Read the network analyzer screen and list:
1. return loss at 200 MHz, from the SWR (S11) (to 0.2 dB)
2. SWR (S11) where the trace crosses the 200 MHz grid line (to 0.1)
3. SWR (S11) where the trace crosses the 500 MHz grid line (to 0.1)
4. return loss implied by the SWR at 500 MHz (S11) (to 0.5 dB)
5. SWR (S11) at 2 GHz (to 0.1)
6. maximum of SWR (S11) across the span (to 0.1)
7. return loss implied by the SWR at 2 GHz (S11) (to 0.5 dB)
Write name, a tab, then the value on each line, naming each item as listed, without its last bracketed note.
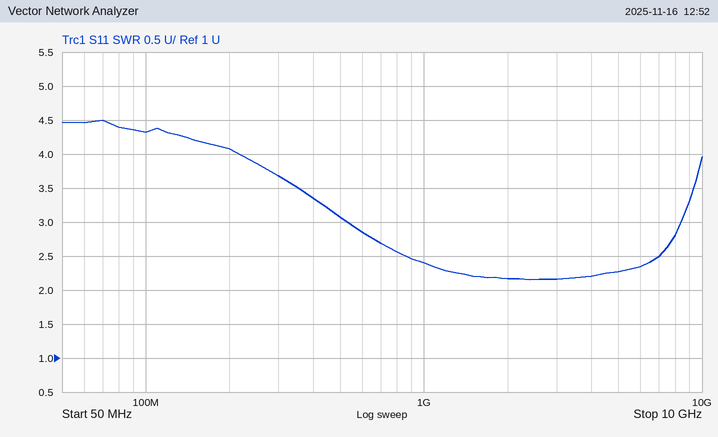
return loss at 200 MHz, from the SWR (S11)	4.4 dB
SWR (S11) where the trace crosses the 200 MHz grid line	4.1
SWR (S11) where the trace crosses the 500 MHz grid line	3.1
return loss implied by the SWR at 500 MHz (S11)	6.0 dB
SWR (S11) at 2 GHz	2.2
maximum of SWR (S11) across the span	4.5
return loss implied by the SWR at 2 GHz (S11)	8.5 dB
